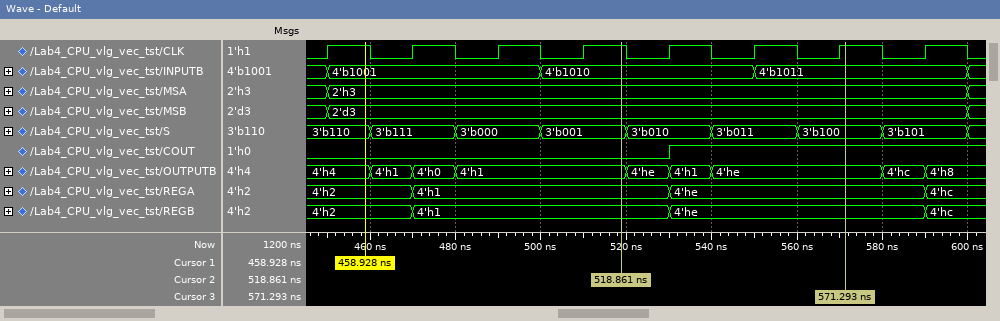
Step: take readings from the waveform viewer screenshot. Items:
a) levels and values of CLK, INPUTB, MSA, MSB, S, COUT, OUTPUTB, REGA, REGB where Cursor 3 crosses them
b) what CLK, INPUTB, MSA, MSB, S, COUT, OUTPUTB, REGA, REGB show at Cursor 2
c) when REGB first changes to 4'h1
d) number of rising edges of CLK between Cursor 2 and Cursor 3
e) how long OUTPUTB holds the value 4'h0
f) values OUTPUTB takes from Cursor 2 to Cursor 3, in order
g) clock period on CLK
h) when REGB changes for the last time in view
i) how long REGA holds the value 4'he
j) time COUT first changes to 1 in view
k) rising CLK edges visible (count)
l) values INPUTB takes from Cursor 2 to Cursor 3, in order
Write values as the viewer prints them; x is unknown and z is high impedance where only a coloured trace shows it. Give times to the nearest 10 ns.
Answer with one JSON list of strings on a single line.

["CLK=1, INPUTB=4'b1011, MSA=2'h3, MSB=2'd3, S=3'b100, COUT=1, OUTPUTB=4'he, REGA=4'he, REGB=4'he", "CLK=1, INPUTB=4'b1010, MSA=2'h3, MSB=2'd3, S=3'b001, COUT=0, OUTPUTB=4'h1, REGA=4'h1, REGB=4'h1", "470 ns", "3", "10 ns", "4'h1, 4'he, 4'h1, 4'he", "20 ns", "590 ns", "60 ns", "530 ns", "8", "4'b1010, 4'b1011"]
